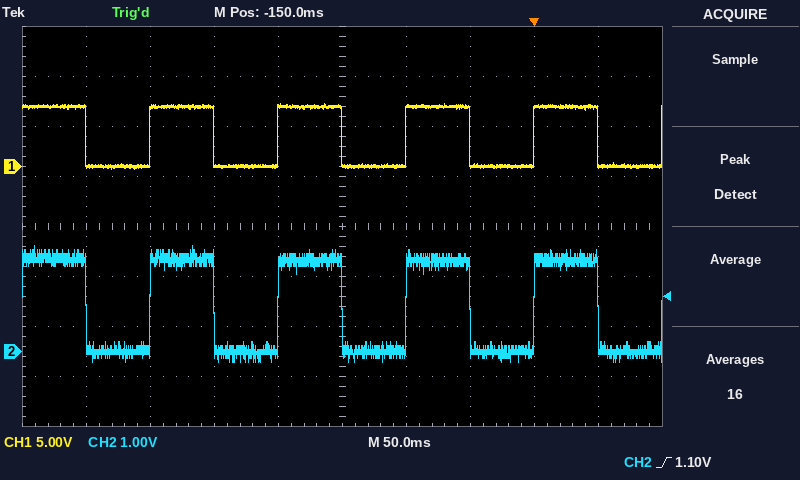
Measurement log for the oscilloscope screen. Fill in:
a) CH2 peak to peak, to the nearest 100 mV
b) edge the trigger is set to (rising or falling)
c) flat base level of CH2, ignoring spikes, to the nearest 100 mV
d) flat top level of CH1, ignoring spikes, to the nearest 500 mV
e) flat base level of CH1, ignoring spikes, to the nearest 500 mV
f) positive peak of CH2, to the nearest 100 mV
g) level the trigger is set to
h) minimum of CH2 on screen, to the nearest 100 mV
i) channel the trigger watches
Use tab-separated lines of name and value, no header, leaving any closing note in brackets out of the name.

CH2 peak to peak, to the nearest 100 mV	2.3 V
edge the trigger is set to	rising
flat base level of CH2, ignoring spikes, to the nearest 100 mV	0.0 V
flat top level of CH1, ignoring spikes, to the nearest 500 mV	6.0 V
flat base level of CH1, ignoring spikes, to the nearest 500 mV	0.0 V
positive peak of CH2, to the nearest 100 mV	2.1 V
level the trigger is set to	1.10 V
minimum of CH2 on screen, to the nearest 100 mV	-200 mV
channel the trigger watches	CH2
